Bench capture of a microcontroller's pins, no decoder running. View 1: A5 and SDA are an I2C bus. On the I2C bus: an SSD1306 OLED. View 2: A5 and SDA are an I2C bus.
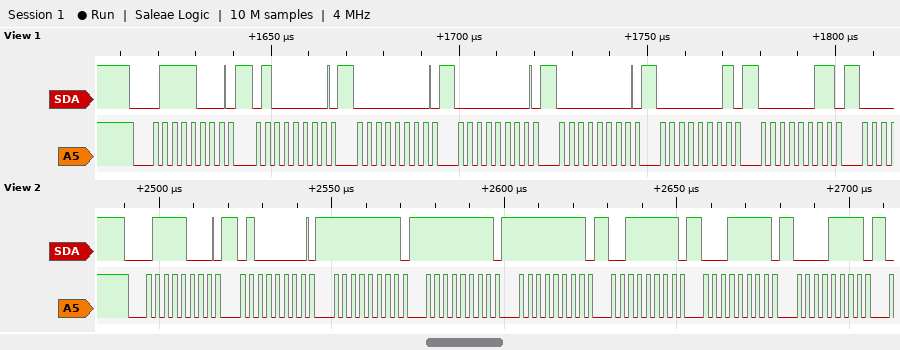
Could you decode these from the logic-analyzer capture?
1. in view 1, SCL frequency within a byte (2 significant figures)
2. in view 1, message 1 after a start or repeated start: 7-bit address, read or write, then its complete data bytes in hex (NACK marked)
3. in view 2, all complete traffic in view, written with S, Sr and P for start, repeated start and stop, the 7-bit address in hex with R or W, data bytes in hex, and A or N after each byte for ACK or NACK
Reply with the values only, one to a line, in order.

400 kHz
0x3C write: 40 00 00 00 01 03
S 3CW A 40 A FF A FF A FF A 3F A 1F A 0F A
